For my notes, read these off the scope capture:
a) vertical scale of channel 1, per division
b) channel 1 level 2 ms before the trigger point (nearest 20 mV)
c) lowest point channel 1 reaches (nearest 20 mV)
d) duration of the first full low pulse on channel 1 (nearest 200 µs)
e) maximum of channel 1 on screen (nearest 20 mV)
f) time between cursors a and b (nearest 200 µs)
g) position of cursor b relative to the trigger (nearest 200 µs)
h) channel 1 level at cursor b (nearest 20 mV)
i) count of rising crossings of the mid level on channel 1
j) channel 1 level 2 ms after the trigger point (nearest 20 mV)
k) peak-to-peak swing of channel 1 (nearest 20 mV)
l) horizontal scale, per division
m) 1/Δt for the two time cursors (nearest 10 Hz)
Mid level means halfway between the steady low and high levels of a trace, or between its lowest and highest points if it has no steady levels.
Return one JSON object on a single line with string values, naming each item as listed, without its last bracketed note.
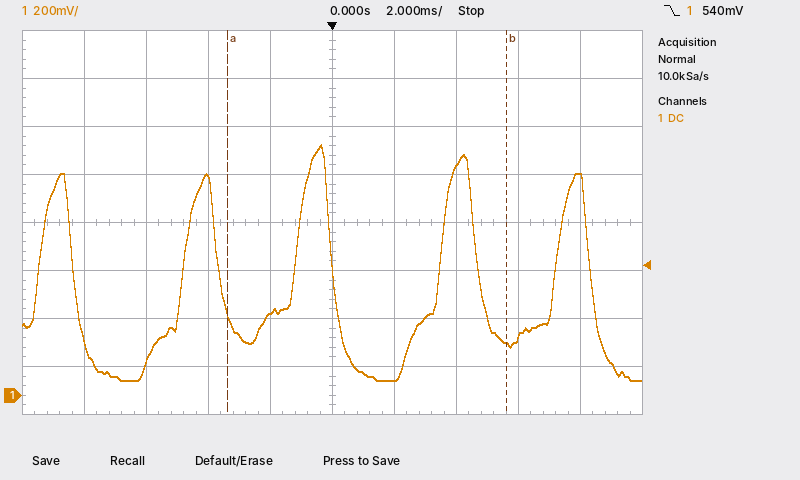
{"vertical scale of channel 1, per division": "200 mV", "channel 1 level 2 ms before the trigger point": "340 mV", "lowest point channel 1 reaches": "60 mV", "duration of the first full low pulse on channel 1": "3.6 ms", "maximum of channel 1 on screen": "1.04 V", "time between cursors a and b": "9.0 ms", "position of cursor b relative to the trigger": "+5.6 ms", "channel 1 level at cursor b": "220 mV", "count of rising crossings of the mid level on channel 1": "5", "channel 1 level 2 ms after the trigger point": "60 mV", "peak-to-peak swing of channel 1": "980 mV", "horizontal scale, per division": "2 ms", "1/Δt for the two time cursors": "110 Hz"}
